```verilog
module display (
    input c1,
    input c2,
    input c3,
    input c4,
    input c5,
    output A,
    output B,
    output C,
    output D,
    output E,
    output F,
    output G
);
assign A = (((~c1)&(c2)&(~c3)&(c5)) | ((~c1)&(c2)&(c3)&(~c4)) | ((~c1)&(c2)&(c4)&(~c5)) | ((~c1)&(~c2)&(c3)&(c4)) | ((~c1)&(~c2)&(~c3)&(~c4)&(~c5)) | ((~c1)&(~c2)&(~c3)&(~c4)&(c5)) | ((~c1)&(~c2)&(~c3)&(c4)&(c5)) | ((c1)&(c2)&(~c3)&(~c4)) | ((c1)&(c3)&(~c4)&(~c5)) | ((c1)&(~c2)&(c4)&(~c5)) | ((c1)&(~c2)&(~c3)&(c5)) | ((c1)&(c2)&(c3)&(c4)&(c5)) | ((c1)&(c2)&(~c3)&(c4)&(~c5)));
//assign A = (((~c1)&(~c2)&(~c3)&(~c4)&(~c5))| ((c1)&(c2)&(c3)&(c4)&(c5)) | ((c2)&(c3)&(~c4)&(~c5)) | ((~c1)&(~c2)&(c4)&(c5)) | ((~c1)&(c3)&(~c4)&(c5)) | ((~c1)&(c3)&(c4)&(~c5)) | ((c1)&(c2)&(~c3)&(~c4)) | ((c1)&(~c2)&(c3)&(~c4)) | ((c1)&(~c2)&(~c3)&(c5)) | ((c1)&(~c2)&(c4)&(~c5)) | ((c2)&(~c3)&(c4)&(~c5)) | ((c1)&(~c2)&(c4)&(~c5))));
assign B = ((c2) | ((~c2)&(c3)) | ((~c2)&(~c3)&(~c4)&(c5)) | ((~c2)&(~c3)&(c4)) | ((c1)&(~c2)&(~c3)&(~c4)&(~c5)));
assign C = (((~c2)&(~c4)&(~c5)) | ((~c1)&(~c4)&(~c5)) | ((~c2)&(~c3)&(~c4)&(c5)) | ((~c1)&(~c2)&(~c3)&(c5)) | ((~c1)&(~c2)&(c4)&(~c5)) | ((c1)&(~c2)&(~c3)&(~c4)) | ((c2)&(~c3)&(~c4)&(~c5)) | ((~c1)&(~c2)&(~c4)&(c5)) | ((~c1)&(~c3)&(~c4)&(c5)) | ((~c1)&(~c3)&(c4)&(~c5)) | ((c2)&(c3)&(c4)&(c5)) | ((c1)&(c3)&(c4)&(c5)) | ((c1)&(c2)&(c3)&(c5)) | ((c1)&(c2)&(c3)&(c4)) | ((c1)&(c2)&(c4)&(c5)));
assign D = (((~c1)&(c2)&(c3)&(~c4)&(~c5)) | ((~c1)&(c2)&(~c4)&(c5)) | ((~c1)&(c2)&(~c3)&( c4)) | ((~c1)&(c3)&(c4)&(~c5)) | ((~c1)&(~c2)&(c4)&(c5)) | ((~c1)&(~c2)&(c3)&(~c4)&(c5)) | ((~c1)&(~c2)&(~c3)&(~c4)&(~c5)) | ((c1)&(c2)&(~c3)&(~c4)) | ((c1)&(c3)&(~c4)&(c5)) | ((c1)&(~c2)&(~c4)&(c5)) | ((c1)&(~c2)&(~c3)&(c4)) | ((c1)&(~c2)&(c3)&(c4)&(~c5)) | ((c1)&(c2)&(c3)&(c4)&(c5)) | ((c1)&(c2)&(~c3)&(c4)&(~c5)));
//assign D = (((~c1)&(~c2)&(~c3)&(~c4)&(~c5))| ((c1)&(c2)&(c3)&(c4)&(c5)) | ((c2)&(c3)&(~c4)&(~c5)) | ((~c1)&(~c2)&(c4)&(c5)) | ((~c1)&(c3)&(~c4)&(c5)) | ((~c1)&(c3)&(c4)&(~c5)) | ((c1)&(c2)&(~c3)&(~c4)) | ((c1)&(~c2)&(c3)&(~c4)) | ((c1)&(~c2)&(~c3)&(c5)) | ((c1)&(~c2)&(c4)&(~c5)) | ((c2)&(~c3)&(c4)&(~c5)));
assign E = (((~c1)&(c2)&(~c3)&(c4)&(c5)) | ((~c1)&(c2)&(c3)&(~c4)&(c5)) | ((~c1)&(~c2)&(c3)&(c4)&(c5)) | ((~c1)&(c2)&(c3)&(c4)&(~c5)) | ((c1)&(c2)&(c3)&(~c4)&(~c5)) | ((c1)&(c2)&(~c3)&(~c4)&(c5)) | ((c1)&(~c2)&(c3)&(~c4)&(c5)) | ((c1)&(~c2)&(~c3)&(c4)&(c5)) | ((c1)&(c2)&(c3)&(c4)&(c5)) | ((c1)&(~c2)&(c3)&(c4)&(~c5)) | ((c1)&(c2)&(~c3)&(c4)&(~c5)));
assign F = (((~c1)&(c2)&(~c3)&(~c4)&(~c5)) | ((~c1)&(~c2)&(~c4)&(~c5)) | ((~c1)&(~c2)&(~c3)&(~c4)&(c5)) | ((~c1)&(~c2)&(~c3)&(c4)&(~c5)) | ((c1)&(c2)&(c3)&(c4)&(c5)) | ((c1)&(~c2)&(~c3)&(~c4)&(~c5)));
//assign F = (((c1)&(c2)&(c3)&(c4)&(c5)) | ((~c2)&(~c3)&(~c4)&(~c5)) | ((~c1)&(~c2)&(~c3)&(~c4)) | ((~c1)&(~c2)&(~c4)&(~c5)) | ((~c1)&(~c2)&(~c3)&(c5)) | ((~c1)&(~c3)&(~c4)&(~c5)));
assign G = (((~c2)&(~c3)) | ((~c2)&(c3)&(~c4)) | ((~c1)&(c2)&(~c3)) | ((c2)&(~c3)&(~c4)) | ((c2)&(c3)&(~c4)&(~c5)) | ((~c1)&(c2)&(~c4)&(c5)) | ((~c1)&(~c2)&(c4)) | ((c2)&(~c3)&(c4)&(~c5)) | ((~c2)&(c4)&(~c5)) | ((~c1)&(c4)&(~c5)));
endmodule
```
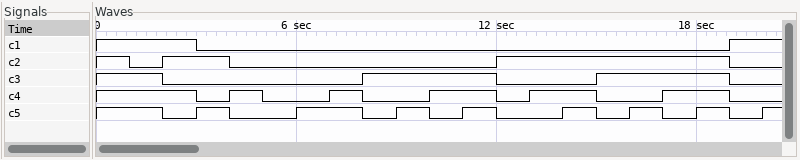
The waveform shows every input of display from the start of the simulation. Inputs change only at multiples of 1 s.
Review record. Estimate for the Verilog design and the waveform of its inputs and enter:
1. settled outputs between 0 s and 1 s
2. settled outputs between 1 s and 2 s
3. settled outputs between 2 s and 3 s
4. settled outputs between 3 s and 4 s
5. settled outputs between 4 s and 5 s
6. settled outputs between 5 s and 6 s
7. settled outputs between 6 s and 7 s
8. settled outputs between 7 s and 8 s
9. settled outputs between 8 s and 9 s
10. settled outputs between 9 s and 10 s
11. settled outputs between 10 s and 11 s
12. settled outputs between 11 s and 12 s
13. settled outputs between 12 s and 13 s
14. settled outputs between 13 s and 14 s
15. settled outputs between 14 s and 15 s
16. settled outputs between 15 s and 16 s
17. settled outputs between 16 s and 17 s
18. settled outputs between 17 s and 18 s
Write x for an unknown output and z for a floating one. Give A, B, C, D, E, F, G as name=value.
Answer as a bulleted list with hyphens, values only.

- A=1, B=1, C=1, D=1, E=1, F=1, G=0
- A=0, B=1, C=1, D=0, E=0, F=0, G=0
- A=1, B=1, C=0, D=1, E=1, F=0, G=1
- A=1, B=1, C=1, D=1, E=0, F=0, G=1
- A=0, B=1, C=1, D=0, E=0, F=1, G=1
- A=1, B=0, C=1, D=1, E=0, F=1, G=1
- A=1, B=1, C=1, D=0, E=0, F=1, G=1
- A=1, B=1, C=1, D=1, E=0, F=0, G=1
- A=0, B=1, C=1, D=0, E=0, F=1, G=1
- A=0, B=1, C=1, D=1, E=0, F=0, G=1
- A=1, B=1, C=1, D=1, E=0, F=0, G=1
- A=1, B=1, C=0, D=1, E=1, F=0, G=1
- A=0, B=1, C=1, D=0, E=0, F=1, G=1
- A=1, B=1, C=1, D=1, E=0, F=0, G=1
- A=1, B=1, C=0, D=1, E=1, F=0, G=1
- A=1, B=1, C=1, D=1, E=0, F=0, G=1
- A=1, B=1, C=0, D=1, E=1, F=0, G=1
- A=1, B=1, C=0, D=1, E=1, F=0, G=1
